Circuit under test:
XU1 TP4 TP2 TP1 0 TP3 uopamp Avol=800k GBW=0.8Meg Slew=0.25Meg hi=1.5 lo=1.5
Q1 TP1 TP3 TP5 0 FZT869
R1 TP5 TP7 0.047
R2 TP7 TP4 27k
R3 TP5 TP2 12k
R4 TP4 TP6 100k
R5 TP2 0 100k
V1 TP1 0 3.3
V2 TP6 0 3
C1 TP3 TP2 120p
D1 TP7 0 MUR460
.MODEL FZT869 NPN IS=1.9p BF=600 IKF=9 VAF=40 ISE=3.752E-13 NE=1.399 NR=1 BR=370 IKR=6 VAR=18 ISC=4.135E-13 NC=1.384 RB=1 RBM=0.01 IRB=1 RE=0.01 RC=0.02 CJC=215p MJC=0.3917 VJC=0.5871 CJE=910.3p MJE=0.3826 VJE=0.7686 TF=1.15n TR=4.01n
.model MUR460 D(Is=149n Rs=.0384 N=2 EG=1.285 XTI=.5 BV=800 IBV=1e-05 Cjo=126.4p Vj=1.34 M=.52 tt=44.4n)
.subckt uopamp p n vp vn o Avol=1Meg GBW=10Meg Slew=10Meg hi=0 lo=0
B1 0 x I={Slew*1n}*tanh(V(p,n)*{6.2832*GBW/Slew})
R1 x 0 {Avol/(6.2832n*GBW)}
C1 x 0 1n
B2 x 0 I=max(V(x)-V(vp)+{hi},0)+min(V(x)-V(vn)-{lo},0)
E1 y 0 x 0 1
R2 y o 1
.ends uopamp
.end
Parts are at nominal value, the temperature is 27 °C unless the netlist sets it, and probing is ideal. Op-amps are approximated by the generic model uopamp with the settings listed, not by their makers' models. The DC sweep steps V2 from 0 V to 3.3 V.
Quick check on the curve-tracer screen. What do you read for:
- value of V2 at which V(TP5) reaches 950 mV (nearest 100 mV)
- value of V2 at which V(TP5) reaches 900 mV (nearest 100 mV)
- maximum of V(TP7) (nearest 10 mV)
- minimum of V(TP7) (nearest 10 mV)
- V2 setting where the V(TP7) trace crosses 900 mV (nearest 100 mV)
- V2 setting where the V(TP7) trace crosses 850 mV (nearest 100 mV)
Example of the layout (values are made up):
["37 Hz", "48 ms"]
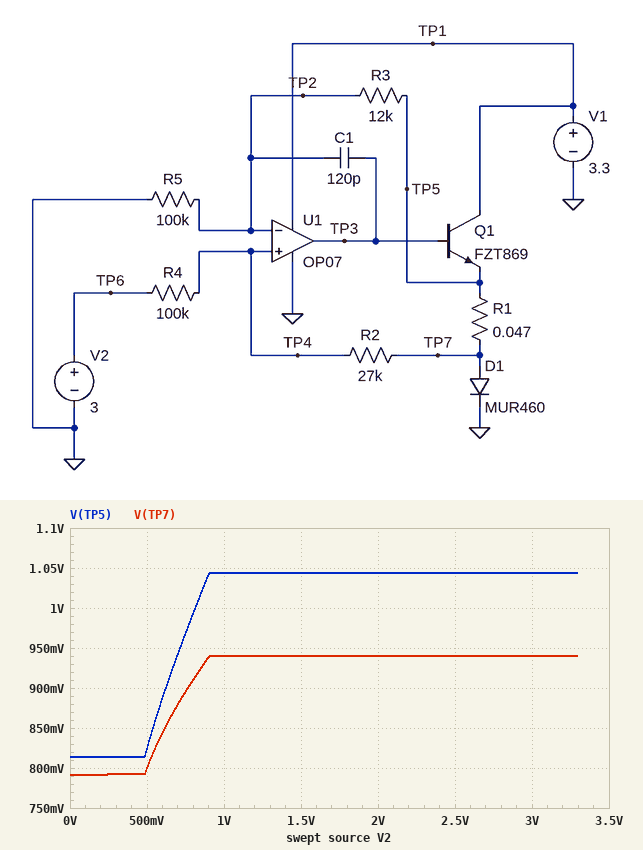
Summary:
["700 mV", "600 mV", "940 mV", "790 mV", "800 mV", "600 mV"]
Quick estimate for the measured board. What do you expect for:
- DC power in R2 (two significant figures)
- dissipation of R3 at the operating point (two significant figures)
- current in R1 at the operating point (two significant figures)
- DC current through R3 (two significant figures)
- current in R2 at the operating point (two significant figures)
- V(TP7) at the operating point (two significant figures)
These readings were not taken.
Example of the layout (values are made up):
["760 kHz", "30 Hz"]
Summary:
["7.1 µW", "1.0 µW", "2.2 A", "9.3 µA", "16 µA", "940 mV"]
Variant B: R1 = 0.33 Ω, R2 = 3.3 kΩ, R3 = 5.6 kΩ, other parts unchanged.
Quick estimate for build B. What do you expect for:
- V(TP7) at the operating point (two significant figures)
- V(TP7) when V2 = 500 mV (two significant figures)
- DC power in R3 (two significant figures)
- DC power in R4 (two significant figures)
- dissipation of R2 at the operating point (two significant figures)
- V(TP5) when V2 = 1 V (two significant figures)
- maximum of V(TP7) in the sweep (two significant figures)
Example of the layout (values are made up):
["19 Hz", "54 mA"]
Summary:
["770 mV", "750 mV", "400 nW", "46 µW", "1.5 µW", "830 mV", "780 mV"]
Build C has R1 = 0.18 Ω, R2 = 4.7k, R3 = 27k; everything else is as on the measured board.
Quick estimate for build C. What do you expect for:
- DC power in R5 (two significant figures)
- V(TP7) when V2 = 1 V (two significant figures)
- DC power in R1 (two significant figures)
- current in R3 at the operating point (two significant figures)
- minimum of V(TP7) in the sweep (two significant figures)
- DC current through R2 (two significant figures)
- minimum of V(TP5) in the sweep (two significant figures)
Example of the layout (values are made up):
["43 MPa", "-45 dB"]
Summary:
["7.2 µW", "870 mV", "250 mW", "8.5 µA", "850 mV", "20 µA", "1.0 V"]
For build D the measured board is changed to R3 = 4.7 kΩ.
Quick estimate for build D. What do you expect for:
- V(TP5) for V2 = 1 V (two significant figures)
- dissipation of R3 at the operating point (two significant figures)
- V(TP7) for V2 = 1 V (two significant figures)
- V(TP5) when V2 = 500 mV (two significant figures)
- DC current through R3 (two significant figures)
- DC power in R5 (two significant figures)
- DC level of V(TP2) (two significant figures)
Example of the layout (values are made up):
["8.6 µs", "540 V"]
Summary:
["950 mV", "470 nW", "890 mV", "810 mV", "10 µA", "9.9 µW", "1.0 V"]
